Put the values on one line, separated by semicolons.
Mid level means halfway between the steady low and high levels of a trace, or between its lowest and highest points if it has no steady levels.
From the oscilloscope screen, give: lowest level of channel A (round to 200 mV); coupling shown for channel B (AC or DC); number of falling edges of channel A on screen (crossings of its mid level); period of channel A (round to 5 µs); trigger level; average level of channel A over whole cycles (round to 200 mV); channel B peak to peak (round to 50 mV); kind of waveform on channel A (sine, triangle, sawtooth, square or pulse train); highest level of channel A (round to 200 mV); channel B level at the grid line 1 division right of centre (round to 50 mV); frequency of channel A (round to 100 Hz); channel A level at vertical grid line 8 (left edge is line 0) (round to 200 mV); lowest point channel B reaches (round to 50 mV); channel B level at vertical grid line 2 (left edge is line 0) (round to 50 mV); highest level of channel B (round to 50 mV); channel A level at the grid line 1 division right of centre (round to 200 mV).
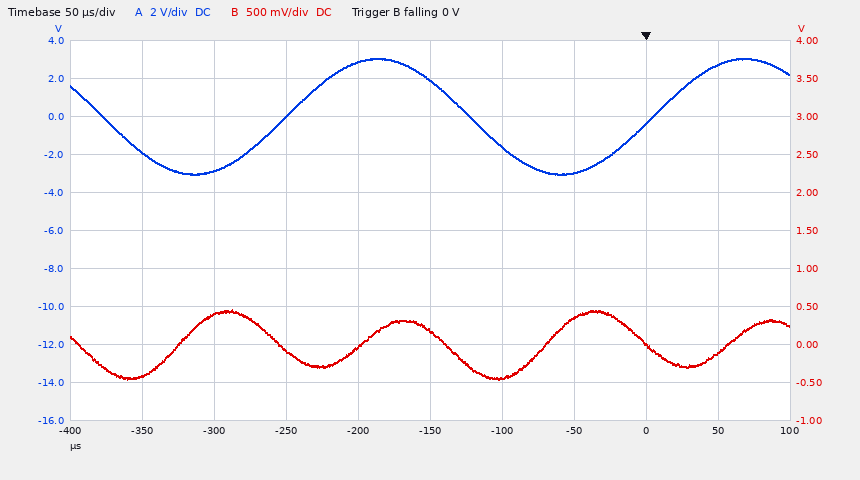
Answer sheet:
-3.0 V; DC; 2; 255 µs; 0 V; 0.0 V; 900 mV; sine; 3.0 V; -450 mV; 3.9 kHz; -400 mV; -450 mV; 400 mV; 450 mV; -1.6 V
